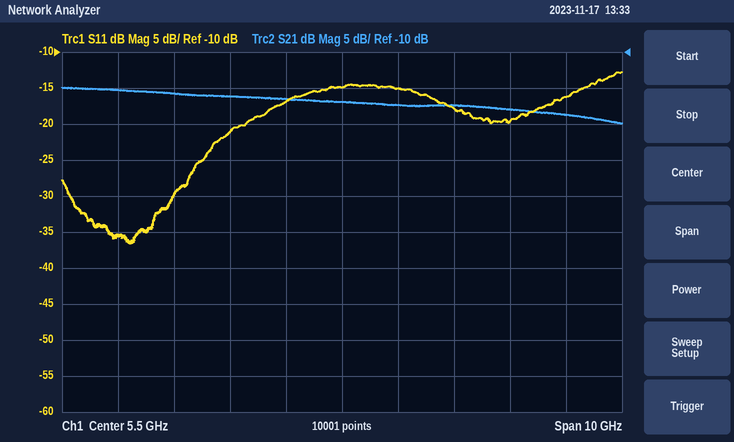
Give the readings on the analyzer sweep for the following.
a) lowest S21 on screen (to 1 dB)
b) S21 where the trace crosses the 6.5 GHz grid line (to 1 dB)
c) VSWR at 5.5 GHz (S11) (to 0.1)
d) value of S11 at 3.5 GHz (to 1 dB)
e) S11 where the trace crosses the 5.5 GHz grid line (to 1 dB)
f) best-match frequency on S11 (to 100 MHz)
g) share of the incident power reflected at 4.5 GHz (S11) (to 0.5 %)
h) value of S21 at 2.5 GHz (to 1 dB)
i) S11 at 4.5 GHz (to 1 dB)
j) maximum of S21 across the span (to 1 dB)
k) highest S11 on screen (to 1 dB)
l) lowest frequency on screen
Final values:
-20 dB
-17 dB
1.4
-21 dB
-15 dB
1.7 GHz
2.0 %
-16 dB
-17 dB
-15 dB
-13 dB
500 MHz
